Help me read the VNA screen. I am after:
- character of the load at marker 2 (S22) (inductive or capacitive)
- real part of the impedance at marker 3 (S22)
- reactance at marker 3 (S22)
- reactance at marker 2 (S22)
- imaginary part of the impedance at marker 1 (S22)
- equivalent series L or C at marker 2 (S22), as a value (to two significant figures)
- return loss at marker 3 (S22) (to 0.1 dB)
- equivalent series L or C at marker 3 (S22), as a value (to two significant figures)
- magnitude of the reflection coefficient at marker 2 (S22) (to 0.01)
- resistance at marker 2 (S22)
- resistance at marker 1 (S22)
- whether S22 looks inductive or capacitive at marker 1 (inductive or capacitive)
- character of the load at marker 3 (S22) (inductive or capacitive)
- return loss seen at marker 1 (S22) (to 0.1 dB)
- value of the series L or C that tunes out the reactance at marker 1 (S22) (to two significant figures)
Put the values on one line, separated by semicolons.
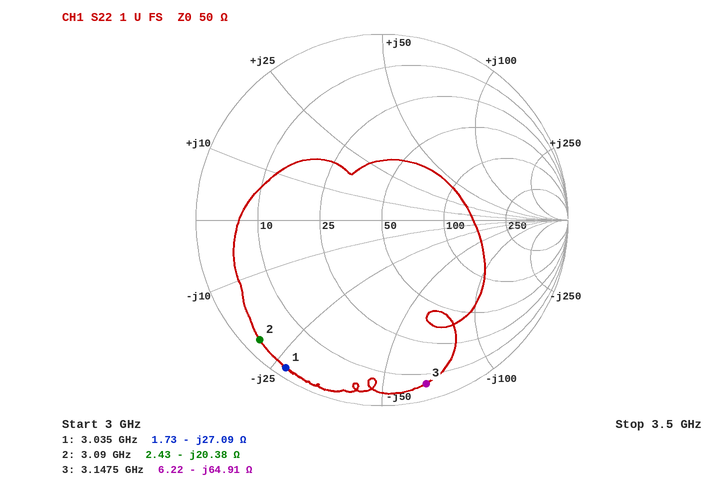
capacitive; 6.22 Ω; -64.91 Ω; -20.38 Ω; -27.09 Ω; 2.5 pF; 0.8 dB; 780 fF; 0.92; 2.43 Ω; 1.73 Ω; capacitive; capacitive; 0.5 dB; 1.4 nH
